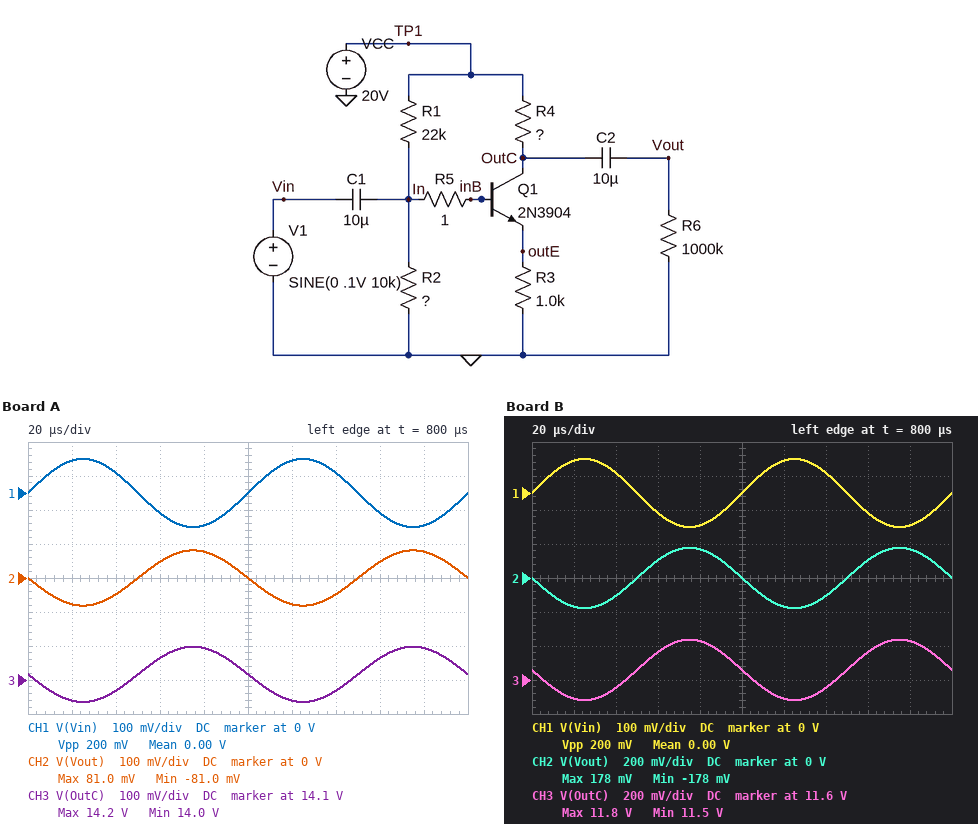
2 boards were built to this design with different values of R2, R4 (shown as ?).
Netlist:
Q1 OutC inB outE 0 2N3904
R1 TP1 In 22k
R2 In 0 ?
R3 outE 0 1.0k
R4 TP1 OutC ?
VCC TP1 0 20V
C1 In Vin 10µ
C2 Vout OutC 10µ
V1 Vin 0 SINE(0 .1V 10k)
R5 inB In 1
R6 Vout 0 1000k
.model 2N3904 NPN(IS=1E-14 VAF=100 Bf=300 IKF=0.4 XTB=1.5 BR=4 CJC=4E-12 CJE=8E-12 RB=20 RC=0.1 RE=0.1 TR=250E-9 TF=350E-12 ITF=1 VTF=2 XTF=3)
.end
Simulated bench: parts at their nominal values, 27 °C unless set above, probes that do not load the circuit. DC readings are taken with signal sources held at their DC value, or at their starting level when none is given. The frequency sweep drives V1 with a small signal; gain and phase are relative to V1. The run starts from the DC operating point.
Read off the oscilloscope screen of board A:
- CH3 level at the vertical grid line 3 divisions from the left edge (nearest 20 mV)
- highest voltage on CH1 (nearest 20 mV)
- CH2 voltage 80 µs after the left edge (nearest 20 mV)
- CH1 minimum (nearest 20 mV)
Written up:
14.16 V
100 mV
80 mV
-100 mV
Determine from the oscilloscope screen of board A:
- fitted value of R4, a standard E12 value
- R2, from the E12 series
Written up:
820 Ω
15 kΩ
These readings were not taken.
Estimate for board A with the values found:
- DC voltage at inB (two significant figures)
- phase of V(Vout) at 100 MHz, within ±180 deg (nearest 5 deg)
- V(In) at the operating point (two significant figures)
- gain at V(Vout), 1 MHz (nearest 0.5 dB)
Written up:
7.9 V
75 deg
7.9 V
-2.0 dB
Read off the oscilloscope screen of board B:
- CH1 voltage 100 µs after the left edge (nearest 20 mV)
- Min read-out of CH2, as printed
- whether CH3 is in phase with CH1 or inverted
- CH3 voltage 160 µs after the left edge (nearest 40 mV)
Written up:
0 V
-178 mV
inverted
11.76 V
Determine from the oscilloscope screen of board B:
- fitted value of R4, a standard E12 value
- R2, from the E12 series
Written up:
1.8 kΩ
8.2 kΩ
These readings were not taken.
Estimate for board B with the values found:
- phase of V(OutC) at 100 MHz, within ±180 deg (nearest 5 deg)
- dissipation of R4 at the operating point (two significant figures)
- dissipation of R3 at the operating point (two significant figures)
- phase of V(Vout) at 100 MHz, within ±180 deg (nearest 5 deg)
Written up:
55 deg
39 mW
22 mW
55 deg
